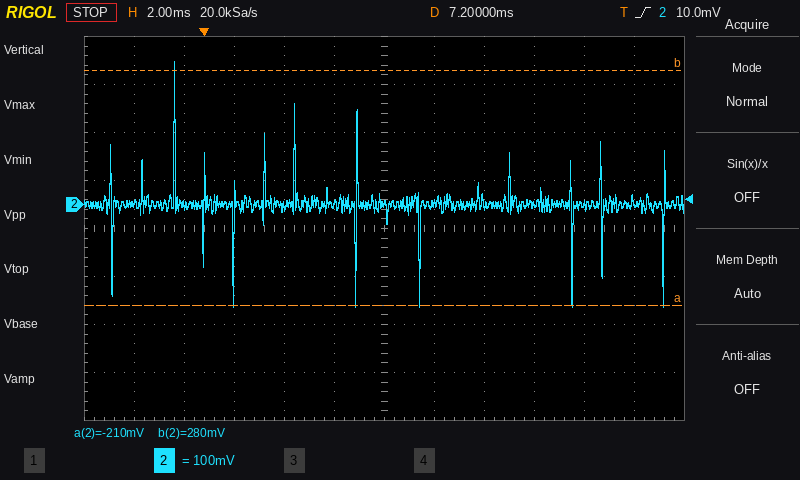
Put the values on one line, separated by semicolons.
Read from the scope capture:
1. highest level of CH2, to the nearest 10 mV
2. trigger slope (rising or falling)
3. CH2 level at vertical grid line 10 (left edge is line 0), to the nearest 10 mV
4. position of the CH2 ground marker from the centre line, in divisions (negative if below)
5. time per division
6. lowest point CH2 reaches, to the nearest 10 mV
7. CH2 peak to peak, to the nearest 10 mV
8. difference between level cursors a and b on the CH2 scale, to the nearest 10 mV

300 mV; rising; 0 mV; +0.5 div; 2 ms; -210 mV; 510 mV; 490 mV
